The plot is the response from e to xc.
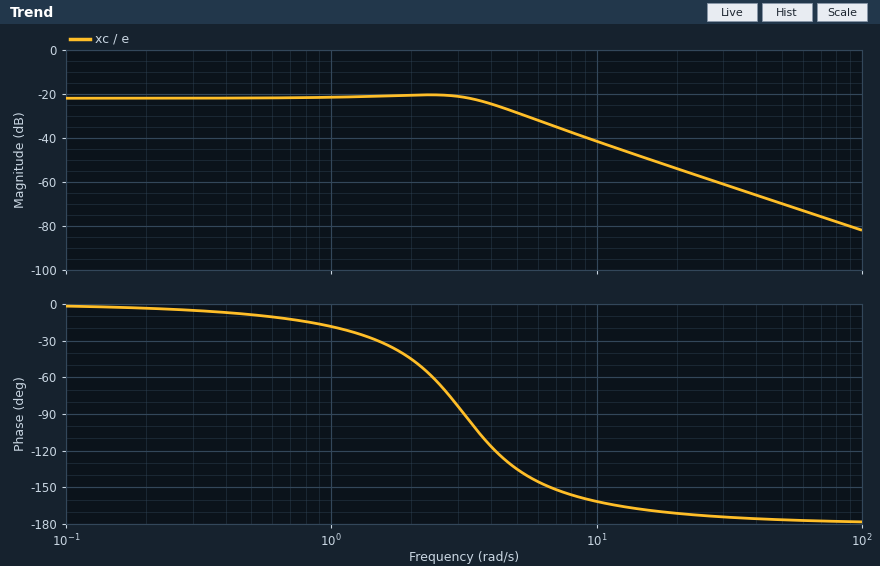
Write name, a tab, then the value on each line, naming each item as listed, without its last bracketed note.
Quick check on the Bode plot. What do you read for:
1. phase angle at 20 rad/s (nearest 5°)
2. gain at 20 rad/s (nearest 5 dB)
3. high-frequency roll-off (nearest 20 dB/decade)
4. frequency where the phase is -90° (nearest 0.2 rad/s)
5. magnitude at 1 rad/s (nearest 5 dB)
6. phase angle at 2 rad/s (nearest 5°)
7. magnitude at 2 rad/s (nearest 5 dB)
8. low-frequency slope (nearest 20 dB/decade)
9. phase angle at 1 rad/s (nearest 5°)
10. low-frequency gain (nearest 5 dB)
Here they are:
phase angle at 20 rad/s	-170°
gain at 20 rad/s	-55 dB
high-frequency roll-off	-40 dB/decade
frequency where the phase is -90°	3.2 rad/s
magnitude at 1 rad/s	-20 dB
phase angle at 2 rad/s	-45°
magnitude at 2 rad/s	-20 dB
low-frequency slope	0 dB/decade
phase angle at 1 rad/s	-20°
low-frequency gain	-20 dB
